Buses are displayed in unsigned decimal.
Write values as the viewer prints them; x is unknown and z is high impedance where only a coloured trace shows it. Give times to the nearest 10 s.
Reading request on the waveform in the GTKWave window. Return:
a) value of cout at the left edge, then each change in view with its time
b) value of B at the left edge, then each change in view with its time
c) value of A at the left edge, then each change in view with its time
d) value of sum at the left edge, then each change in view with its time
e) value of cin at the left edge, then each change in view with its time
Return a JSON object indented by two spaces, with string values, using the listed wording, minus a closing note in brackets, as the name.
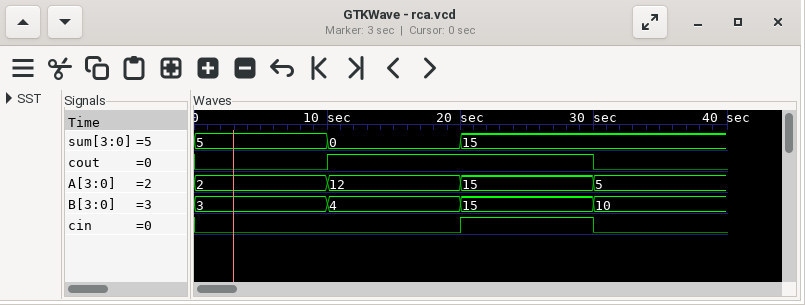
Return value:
{
  "value of cout at the left edge, then each change in view with its time": "0, 1 at 10 s, 0 at 30 s",
  "value of B at the left edge, then each change in view with its time": "3, 4 at 10 s, 15 at 20 s, 10 at 30 s",
  "value of A at the left edge, then each change in view with its time": "2, 12 at 10 s, 15 at 20 s, 5 at 30 s",
  "value of sum at the left edge, then each change in view with its time": "5, 0 at 10 s, 15 at 20 s",
  "value of cin at the left edge, then each change in view with its time": "0, 1 at 20 s, 0 at 30 s"
}
